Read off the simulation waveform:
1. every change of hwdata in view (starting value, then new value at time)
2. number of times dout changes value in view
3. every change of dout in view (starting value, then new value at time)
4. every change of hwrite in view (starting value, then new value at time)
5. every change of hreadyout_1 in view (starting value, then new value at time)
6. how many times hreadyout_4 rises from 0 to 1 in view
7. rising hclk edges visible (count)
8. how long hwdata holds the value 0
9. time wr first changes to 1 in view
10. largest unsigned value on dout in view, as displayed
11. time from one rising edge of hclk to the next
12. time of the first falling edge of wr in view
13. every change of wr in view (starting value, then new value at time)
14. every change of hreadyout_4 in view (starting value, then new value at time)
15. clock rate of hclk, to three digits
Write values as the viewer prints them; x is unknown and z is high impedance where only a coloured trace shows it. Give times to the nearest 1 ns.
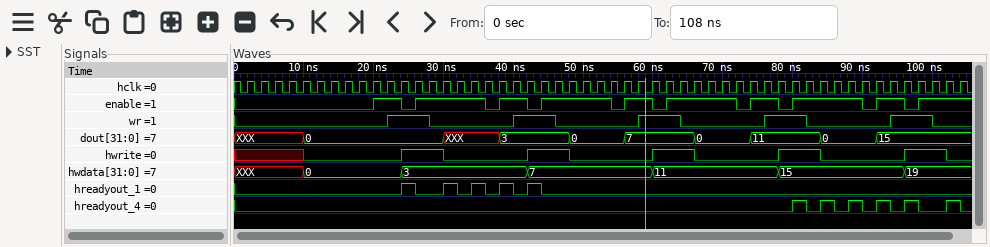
XXX, 0 at 10 ns, 3 at 24 ns, 7 at 42 ns, 11 at 60 ns, 15 at 78 ns, 19 at 96 ns
9
XXX, 0 at 10 ns, XXX at 30 ns, 3 at 38 ns, 0 at 48 ns, 7 at 56 ns, 0 at 66 ns, 11 at 74 ns, 0 at 84 ns, 15 at 92 ns
x, 0 at 10 ns, 1 at 24 ns, 0 at 30 ns, 1 at 42 ns, 0 at 48 ns, 1 at 60 ns, 0 at 66 ns, 1 at 78 ns, 0 at 84 ns, 1 at 96 ns, 0 at 102 ns
0, 1 at 24 ns, 0 at 26 ns, 1 at 30 ns, 0 at 32 ns, 1 at 34 ns, 0 at 36 ns, 1 at 38 ns, 0 at 40 ns, 1 at 42 ns, 0 at 44 ns
6
52
14 ns
22 ns
15
2 ns
28 ns
0, 1 at 22 ns, 0 at 28 ns, 1 at 40 ns, 0 at 46 ns, 1 at 58 ns, 0 at 64 ns, 1 at 76 ns, 0 at 82 ns, 1 at 94 ns, 0 at 100 ns
0, 1 at 80 ns, 0 at 82 ns, 1 at 84 ns, 0 at 86 ns, 1 at 88 ns, 0 at 90 ns, 1 at 92 ns, 0 at 94 ns, 1 at 96 ns, 0 at 98 ns, 1 at 102 ns, 0 at 104 ns
500 MHz
